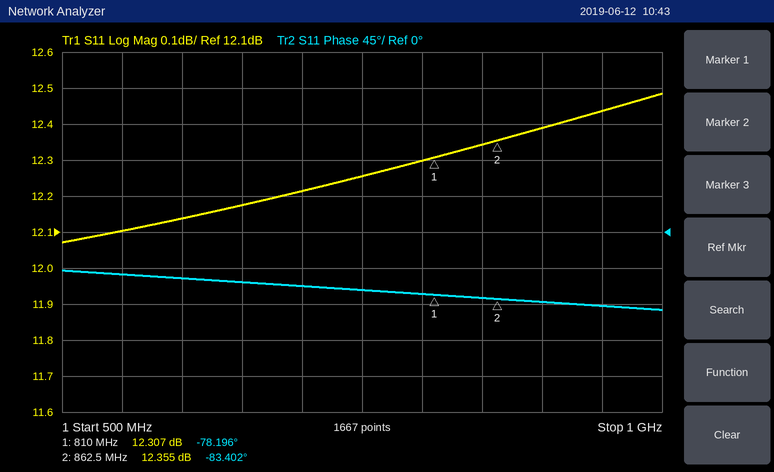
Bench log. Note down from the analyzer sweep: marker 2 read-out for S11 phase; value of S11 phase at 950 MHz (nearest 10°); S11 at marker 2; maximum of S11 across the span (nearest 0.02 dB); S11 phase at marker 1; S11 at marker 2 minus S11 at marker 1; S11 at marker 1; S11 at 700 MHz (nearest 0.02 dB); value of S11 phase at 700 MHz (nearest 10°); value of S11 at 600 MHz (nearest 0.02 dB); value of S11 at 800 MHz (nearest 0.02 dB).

-83.402°
-90°
12.355 dB
12.48 dB
-78.196°
0.048 dB
12.307 dB
12.22 dB
-70°
12.14 dB
12.30 dB
